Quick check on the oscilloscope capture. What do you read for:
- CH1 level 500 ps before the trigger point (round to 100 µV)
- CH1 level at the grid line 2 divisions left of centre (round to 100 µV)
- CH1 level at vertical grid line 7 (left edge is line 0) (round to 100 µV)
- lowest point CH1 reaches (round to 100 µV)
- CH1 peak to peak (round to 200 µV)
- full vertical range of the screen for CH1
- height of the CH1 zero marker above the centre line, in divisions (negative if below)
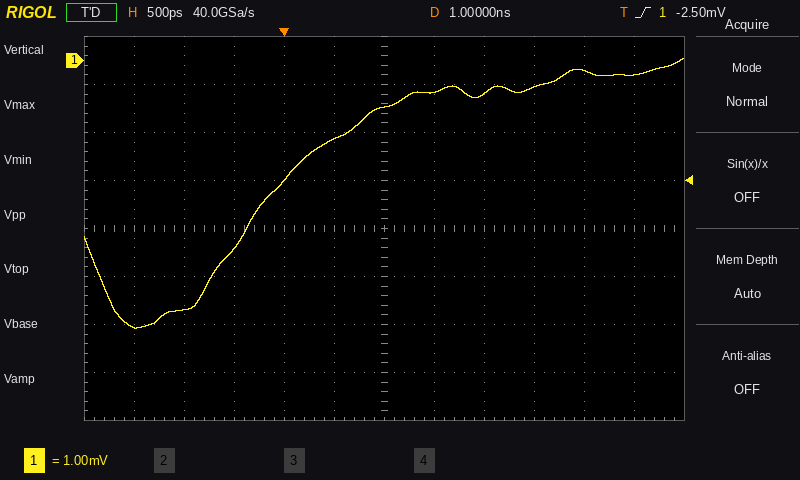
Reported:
-3.9 mV
-2.5 mV
-700 µV
-5.6 mV
5.6 mV
8 mV
+3.5 div
